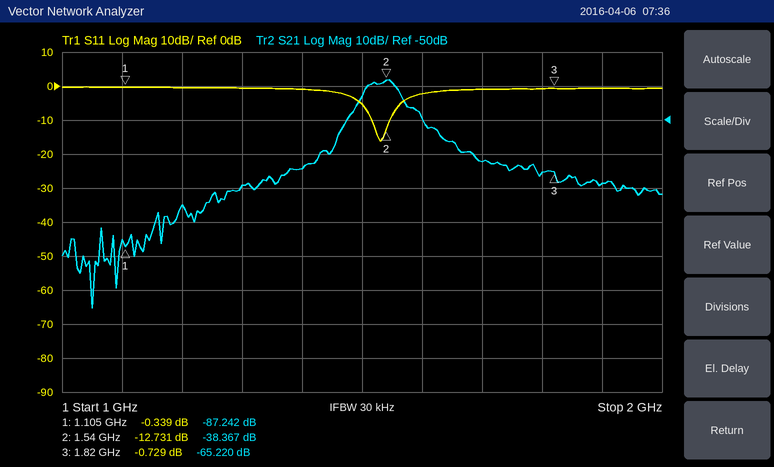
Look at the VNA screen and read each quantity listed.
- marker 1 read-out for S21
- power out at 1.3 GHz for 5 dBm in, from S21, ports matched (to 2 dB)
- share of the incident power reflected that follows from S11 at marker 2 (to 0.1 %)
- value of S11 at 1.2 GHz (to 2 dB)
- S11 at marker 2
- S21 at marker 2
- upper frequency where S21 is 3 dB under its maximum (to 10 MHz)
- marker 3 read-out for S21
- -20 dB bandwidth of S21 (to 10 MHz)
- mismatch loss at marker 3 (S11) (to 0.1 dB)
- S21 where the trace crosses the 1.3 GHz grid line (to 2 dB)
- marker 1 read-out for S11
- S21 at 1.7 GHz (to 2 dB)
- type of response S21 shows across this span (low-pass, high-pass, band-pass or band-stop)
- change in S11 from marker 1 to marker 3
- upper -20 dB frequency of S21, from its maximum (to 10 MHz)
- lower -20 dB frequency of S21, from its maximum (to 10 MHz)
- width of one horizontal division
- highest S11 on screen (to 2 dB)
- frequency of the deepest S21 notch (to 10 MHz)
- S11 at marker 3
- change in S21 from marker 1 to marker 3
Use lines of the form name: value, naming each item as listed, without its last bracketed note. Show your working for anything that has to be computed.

marker 1 read-out for S21: -87.242 dB
power out at 1.3 GHz for 5 dBm in, from S21, ports matched: 5 dBm + (-70 dB) = -64 dBm
share of the incident power reflected that follows from S11 at marker 2: 10^(-12.731/10) ≈ 5.3 %
value of S11 at 1.2 GHz: 0 dB
S11 at marker 2: -12.731 dB
S21 at marker 2: -38.367 dB
upper frequency where S21 is 3 dB under its maximum: 1.56 GHz
marker 3 read-out for S21: -65.220 dB
-20 dB bandwidth of S21: 1.66 GHz − 1.45 GHz = 210 MHz
mismatch loss at marker 3 (S11): −10 log10(1 − 10^(-0.729/10)) ≈ 8.1 dB
S21 where the trace crosses the 1.3 GHz grid line: -70 dB
marker 1 read-out for S11: -0.339 dB
S21 at 1.7 GHz: -62 dB
type of response S21 shows across this span: band-pass
change in S11 from marker 1 to marker 3: -0.729 − (-0.339) = -0.390 dB
upper -20 dB frequency of S21, from its maximum: 1.66 GHz
lower -20 dB frequency of S21, from its maximum: 1.45 GHz
width of one horizontal division: 100 MHz
highest S11 on screen: 0 dB
frequency of the deepest S21 notch: 1.05 GHz
S11 at marker 3: -0.729 dB
change in S21 from marker 1 to marker 3: -65.22 − (-87.242) = 22.022 dB
